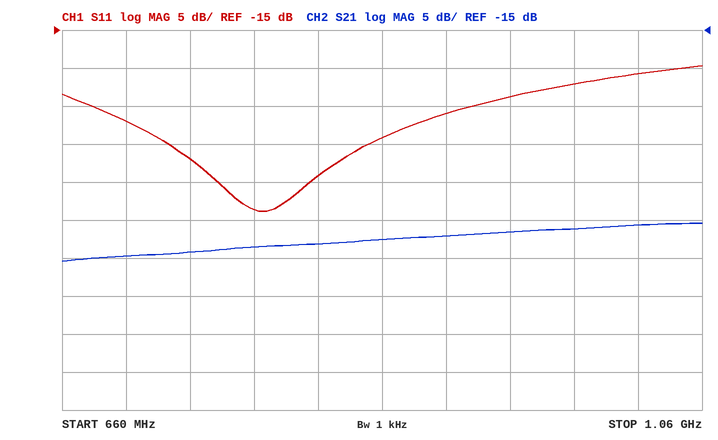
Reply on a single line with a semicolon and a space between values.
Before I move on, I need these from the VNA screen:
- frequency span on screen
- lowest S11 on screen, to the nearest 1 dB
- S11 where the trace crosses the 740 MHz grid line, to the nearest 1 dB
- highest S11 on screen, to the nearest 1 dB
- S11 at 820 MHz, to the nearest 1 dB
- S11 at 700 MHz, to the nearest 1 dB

400 MHz; -39 dB; -32 dB; -20 dB; -34 dB; -27 dB
